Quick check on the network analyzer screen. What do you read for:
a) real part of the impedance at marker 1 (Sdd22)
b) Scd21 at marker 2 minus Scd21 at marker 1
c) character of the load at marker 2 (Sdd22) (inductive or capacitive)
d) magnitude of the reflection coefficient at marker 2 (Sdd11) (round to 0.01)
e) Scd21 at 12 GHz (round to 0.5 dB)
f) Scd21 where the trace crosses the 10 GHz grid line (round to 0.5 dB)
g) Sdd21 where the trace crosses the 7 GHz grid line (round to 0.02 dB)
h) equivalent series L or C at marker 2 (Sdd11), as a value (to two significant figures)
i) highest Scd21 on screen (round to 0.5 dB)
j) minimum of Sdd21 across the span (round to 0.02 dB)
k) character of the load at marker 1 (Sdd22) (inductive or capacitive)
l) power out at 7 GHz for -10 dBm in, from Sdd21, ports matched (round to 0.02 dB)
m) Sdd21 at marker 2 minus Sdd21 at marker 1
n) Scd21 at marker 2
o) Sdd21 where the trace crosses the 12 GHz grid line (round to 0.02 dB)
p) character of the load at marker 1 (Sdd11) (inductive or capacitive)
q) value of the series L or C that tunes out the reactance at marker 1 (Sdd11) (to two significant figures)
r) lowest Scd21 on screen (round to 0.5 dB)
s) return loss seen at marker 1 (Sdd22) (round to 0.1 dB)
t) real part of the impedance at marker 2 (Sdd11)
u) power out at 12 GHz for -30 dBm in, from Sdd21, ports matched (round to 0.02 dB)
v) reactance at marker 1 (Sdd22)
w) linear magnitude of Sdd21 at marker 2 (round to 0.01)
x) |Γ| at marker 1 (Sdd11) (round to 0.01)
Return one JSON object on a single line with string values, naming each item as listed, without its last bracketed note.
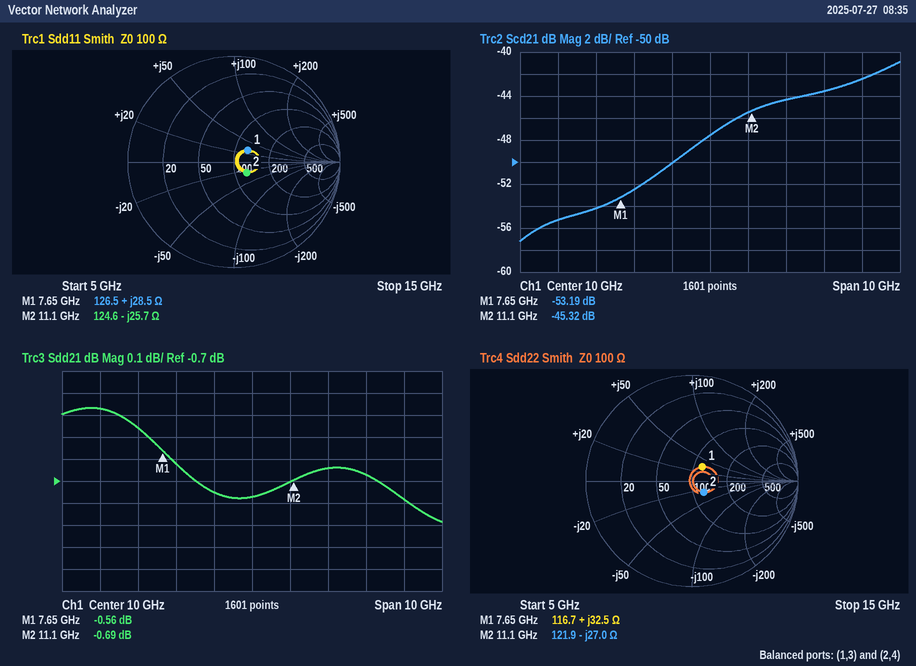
{"real part of the impedance at marker 1": "116.7 Ω", "Scd21 at marker 2 minus Scd21 at marker 1": "7.87 dB", "character of the load at marker 2 (Sdd22)": "capacitive", "magnitude of the reflection coefficient at marker 2 (Sdd11)": "0.16", "Scd21 at 12 GHz": "-44.5 dB", "Scd21 where the trace crosses the 10 GHz grid line": "-47.5 dB", "Sdd21 where the trace crosses the 7 GHz grid line": "-0.46 dB", "equivalent series L or C at marker 2 (Sdd11), as a value": "560 fF", "highest Scd21 on screen": "-41.0 dB", "minimum of Sdd21 across the span": "-0.88 dB", "character of the load at marker 1 (Sdd22)": "inductive", "power out at 7 GHz for -10 dBm in, from Sdd21, ports matched": "-10.46 dBm", "Sdd21 at marker 2 minus Sdd21 at marker 1": "-0.13 dB", "Scd21 at marker 2": "-45.32 dB", "Sdd21 where the trace crosses the 12 GHz grid line": "-0.64 dB", "character of the load at marker 1 (Sdd11)": "inductive", "value of the series L or C that tunes out the reactance at marker 1 (Sdd11)": "730 fF", "lowest Scd21 on screen": "-57.0 dB", "return loss seen at marker 1 (Sdd22)": "15.6 dB", "real part of the impedance at marker 2": "124.6 Ω", "power out at 12 GHz for -30 dBm in, from Sdd21, ports matched": "-30.64 dBm", "reactance at marker 1": "+32.5 Ω", "linear magnitude of Sdd21 at marker 2": "0.92", "|Γ| at marker 1 (Sdd11)": "0.17"}
